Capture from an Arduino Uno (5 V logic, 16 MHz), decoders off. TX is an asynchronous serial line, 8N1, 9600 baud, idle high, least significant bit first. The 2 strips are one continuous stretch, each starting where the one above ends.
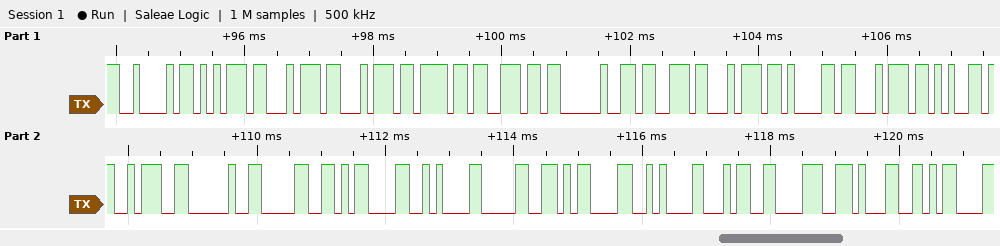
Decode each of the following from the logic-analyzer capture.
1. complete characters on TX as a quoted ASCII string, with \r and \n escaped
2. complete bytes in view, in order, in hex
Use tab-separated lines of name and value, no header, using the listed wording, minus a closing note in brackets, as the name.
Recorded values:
complete characters on TX as a quoted ASCII string, with \r and \n escaped	"Button state: 0\r\n0\r\n481\r"
complete bytes in view, in order, in hex	42 75 74 74 6F 6E 20 73 74 61 74 65 3A 20 30 0D 0A 30 0D 0A 34 38 31 0D
